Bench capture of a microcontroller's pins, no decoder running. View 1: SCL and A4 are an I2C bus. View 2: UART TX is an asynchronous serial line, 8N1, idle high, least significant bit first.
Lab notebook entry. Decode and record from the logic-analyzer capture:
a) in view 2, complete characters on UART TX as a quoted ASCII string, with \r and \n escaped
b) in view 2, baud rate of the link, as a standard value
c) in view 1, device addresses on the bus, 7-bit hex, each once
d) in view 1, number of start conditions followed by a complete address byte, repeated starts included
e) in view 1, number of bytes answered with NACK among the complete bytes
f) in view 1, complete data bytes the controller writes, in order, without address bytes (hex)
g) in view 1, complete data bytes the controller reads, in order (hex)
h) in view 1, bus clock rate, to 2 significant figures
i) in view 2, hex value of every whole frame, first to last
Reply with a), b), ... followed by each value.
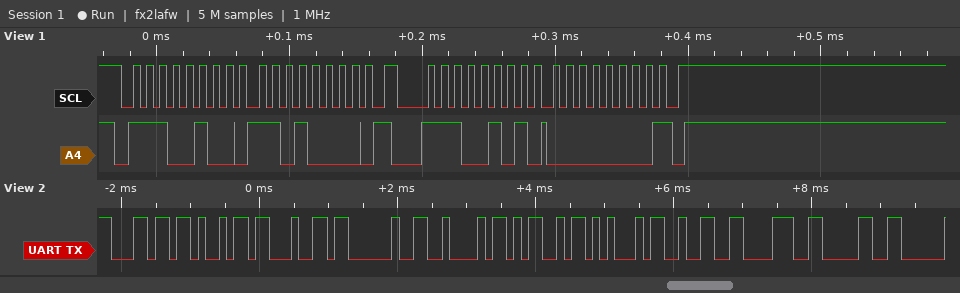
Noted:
a) "lid BME280"
b) 9600 baud
c) 0x72
d) 2
e) 1
f) D0
g) 00
h) 100 kHz
i) 6C 69 64 20 42 4D 45 32 38 30
